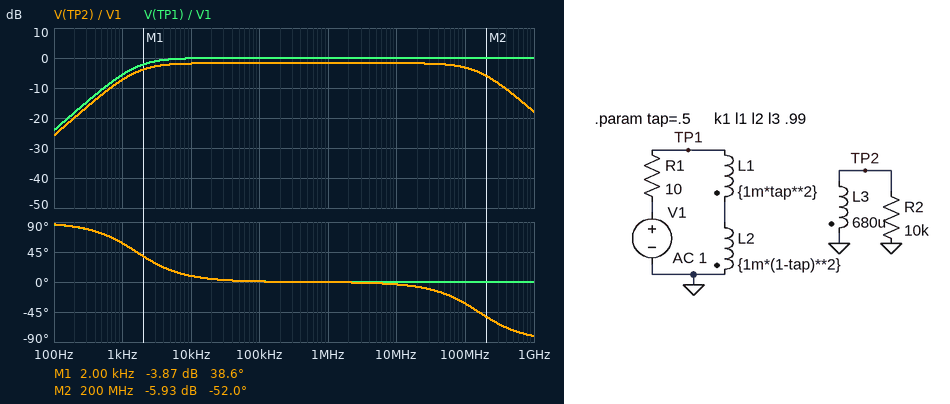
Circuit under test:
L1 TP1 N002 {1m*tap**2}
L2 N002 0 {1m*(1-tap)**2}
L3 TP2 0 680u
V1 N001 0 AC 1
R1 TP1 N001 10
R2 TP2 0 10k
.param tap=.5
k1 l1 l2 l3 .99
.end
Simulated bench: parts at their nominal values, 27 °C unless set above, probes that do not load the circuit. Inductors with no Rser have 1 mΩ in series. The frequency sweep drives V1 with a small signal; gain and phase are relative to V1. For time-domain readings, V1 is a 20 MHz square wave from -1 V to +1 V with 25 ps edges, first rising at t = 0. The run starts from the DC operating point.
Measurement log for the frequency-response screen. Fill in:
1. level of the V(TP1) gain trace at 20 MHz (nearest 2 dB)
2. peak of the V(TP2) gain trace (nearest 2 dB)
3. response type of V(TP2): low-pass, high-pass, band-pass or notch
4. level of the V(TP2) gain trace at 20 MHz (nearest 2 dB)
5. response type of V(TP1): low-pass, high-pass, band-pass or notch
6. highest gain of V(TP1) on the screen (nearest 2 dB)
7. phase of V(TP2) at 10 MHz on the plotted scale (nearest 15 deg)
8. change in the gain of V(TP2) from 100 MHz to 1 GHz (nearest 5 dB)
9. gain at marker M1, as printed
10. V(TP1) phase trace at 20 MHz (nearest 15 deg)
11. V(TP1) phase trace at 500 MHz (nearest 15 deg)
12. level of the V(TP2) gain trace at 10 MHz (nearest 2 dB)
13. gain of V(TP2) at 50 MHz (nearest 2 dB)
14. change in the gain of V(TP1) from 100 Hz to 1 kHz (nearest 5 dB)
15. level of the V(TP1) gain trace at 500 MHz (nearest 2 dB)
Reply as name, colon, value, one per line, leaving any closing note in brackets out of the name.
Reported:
level of the V(TP1) gain trace at 20 MHz: 0 dB
peak of the V(TP2) gain trace: -2 dB
response type of V(TP2): low-pass, high-pass, band-pass or notch: band-pass
level of the V(TP2) gain trace at 20 MHz: -2 dB
response type of V(TP1): low-pass, high-pass, band-pass or notch: high-pass
highest gain of V(TP1) on the screen: 0 dB
phase of V(TP2) at 10 MHz on the plotted scale: 0 deg
change in the gain of V(TP2) from 100 MHz to 1 GHz: -15 dB
gain at marker M1, as printed: -3.87 dB
V(TP1) phase trace at 20 MHz: 0 deg
V(TP1) phase trace at 500 MHz: 0 deg
level of the V(TP2) gain trace at 10 MHz: -2 dB
gain of V(TP2) at 50 MHz: -2 dB
change in the gain of V(TP1) from 100 Hz to 1 kHz: 20 dB
level of the V(TP1) gain trace at 500 MHz: 0 dB
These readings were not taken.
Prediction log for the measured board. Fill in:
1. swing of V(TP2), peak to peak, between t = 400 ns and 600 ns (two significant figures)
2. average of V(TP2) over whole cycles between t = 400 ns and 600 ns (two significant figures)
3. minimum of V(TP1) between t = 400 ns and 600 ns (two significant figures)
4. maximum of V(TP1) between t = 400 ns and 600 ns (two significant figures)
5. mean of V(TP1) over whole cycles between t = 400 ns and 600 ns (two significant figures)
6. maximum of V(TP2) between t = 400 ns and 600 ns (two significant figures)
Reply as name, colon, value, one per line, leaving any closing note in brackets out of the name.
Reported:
swing of V(TP2), peak to peak, between t = 400 ns and 600 ns: 1.6 V
average of V(TP2) over whole cycles between t = 400 ns and 600 ns: 820 mV
minimum of V(TP1) between t = 400 ns and 600 ns: -7.5 mV
maximum of V(TP1) between t = 400 ns and 600 ns: 2.0 V
mean of V(TP1) over whole cycles between t = 400 ns and 600 ns: 990 mV
maximum of V(TP2) between t = 400 ns and 600 ns: 1.6 V
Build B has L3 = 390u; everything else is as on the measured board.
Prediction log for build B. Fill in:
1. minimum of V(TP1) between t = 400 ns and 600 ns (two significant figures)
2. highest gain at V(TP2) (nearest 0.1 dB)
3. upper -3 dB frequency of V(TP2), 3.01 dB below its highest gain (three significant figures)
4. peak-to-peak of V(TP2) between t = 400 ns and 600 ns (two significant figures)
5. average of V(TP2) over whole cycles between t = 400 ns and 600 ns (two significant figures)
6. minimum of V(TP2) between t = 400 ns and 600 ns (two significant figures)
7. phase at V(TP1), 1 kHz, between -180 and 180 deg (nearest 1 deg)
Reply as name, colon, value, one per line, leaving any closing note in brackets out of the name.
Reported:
minimum of V(TP1) between t = 400 ns and 600 ns: -7.0 mV
highest gain at V(TP2): -4.1 dB
upper -3 dB frequency of V(TP2), 3.01 dB below its highest gain: 273 MHz
peak-to-peak of V(TP2) between t = 400 ns and 600 ns: 1.2 V
average of V(TP2) over whole cycles between t = 400 ns and 600 ns: 620 mV
minimum of V(TP2) between t = 400 ns and 600 ns: -3.7 mV
phase at V(TP1), 1 kHz, between -180 and 180 deg: 58 deg
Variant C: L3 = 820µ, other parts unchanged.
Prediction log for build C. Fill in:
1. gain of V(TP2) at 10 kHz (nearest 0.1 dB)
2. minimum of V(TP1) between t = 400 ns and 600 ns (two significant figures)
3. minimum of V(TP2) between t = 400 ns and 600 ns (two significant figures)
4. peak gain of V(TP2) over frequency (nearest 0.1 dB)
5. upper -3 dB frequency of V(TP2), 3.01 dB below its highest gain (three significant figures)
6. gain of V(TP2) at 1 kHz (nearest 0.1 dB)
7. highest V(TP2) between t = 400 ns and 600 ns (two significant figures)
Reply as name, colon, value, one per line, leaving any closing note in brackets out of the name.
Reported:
gain of V(TP2) at 10 kHz: -1.0 dB
minimum of V(TP1) between t = 400 ns and 600 ns: -7.8 mV
minimum of V(TP2) between t = 400 ns and 600 ns: -5.4 mV
peak gain of V(TP2) over frequency: -0.9 dB
upper -3 dB frequency of V(TP2), 3.01 dB below its highest gain: 130 MHz
gain of V(TP2) at 1 kHz: -6.4 dB
highest V(TP2) between t = 400 ns and 600 ns: 1.8 V
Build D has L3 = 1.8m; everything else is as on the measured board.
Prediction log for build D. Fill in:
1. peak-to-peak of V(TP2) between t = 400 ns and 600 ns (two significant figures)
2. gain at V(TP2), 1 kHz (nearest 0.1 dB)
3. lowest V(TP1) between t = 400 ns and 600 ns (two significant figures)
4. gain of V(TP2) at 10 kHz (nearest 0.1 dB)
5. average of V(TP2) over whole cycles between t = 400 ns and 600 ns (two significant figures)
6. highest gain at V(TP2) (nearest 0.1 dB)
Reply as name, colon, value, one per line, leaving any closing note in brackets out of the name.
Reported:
peak-to-peak of V(TP2) between t = 400 ns and 600 ns: 2.7 V
gain at V(TP2), 1 kHz: -3.0 dB
lowest V(TP1) between t = 400 ns and 600 ns: -9.7 mV
gain of V(TP2) at 10 kHz: 2.4 dB
average of V(TP2) over whole cycles between t = 400 ns and 600 ns: 1.3 V
highest gain at V(TP2): 2.5 dB
